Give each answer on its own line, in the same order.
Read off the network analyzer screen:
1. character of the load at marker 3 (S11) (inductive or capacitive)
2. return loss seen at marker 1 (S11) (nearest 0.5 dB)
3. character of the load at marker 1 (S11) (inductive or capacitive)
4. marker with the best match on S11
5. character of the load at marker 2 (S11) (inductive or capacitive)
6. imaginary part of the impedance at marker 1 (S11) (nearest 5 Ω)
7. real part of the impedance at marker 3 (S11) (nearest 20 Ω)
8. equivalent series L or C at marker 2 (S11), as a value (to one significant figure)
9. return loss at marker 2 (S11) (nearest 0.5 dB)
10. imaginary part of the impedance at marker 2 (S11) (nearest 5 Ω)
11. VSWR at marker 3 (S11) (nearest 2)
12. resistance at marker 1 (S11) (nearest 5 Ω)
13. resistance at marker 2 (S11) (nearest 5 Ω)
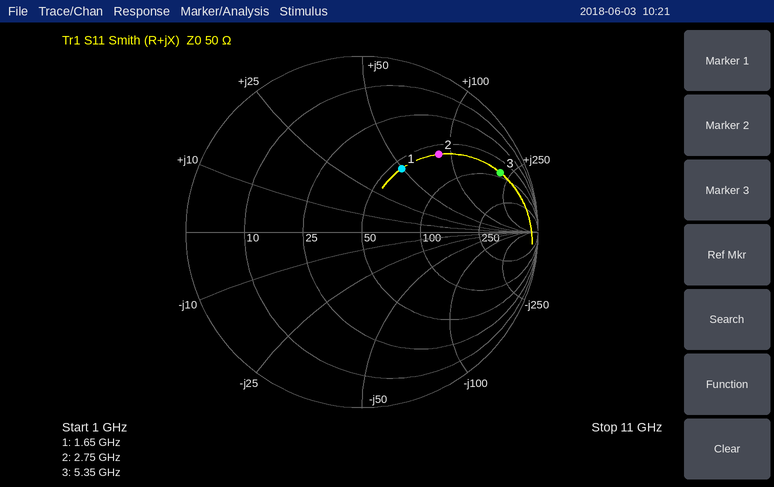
inductive
7.5 dB
inductive
marker 1
inductive
+50 Ω
80 Ω
5 nH
4.0 dB
+85 Ω
12
55 Ω
60 Ω
